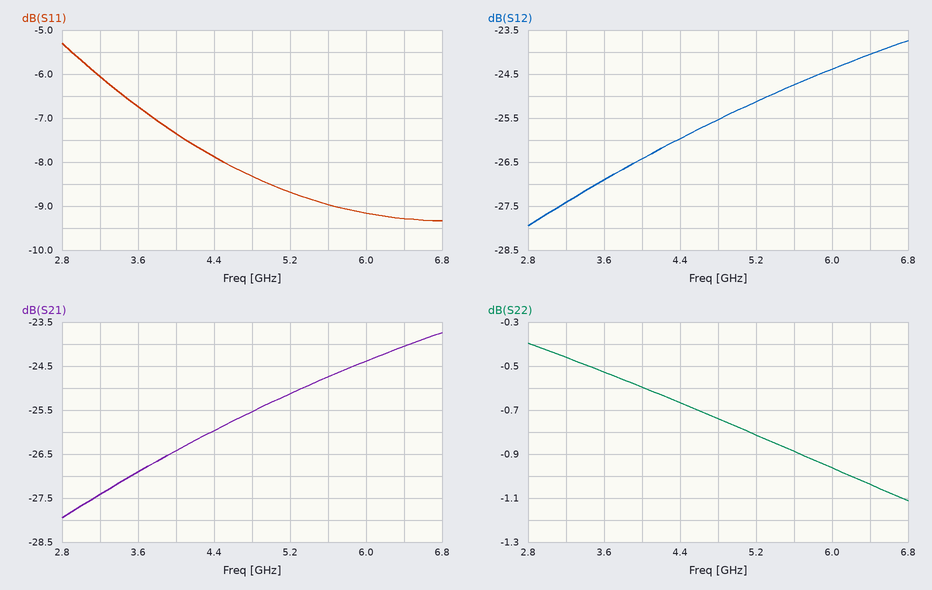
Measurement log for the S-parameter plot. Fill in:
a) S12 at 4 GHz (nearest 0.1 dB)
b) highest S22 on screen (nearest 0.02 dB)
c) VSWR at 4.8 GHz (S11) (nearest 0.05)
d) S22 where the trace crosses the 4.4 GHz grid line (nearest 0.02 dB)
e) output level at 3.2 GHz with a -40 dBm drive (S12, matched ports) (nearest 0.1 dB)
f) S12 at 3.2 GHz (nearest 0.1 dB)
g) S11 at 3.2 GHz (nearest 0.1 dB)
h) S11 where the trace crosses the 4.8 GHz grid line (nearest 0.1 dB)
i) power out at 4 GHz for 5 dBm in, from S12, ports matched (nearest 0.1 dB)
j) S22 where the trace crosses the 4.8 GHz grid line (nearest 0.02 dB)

-26.4 dB
-0.40 dB
2.25
-0.66 dB
-67.4 dBm
-27.4 dB
-6.1 dB
-8.3 dB
-21.4 dBm
-0.74 dB
